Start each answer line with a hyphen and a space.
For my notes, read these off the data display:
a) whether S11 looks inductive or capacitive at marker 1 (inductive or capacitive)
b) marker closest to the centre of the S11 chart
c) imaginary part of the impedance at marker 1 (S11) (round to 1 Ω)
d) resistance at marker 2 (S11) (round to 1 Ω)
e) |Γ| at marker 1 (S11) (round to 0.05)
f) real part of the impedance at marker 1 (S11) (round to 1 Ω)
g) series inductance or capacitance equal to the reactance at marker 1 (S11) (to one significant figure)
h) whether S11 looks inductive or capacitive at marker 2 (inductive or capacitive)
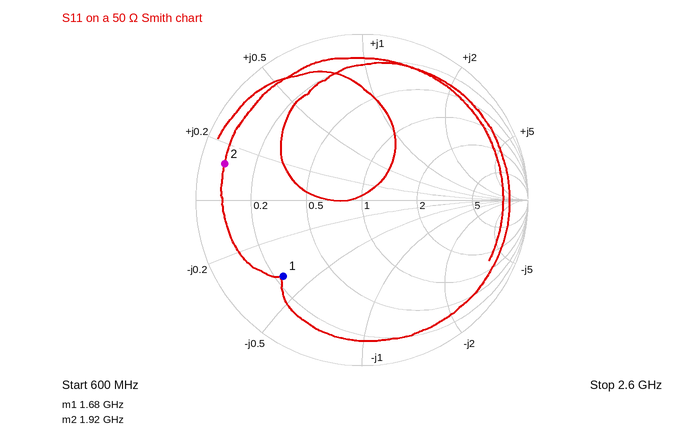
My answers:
- capacitive
- marker 1
- -19 Ω
- 4 Ω
- 0.65
- 12 Ω
- 5 pF
- inductive
